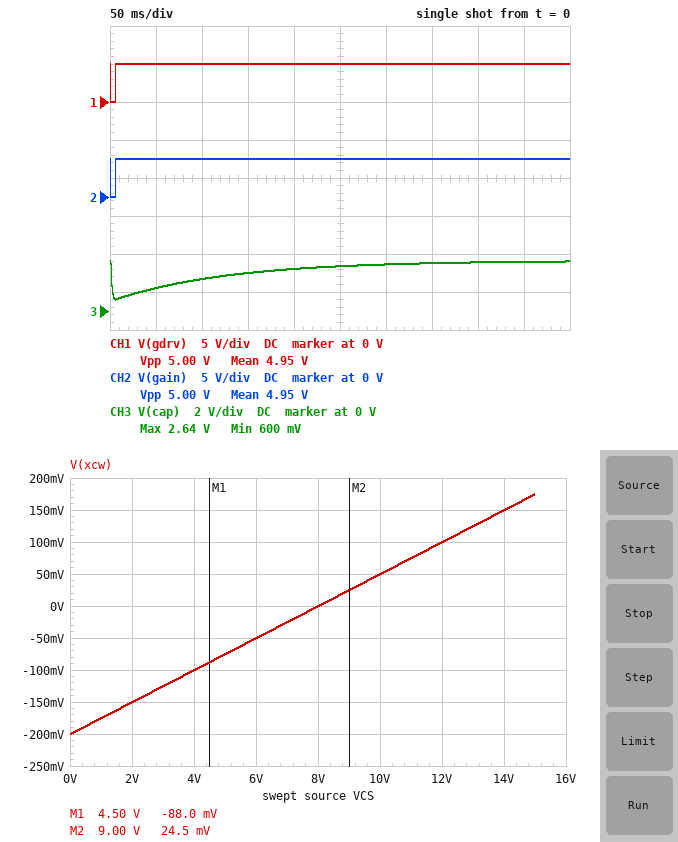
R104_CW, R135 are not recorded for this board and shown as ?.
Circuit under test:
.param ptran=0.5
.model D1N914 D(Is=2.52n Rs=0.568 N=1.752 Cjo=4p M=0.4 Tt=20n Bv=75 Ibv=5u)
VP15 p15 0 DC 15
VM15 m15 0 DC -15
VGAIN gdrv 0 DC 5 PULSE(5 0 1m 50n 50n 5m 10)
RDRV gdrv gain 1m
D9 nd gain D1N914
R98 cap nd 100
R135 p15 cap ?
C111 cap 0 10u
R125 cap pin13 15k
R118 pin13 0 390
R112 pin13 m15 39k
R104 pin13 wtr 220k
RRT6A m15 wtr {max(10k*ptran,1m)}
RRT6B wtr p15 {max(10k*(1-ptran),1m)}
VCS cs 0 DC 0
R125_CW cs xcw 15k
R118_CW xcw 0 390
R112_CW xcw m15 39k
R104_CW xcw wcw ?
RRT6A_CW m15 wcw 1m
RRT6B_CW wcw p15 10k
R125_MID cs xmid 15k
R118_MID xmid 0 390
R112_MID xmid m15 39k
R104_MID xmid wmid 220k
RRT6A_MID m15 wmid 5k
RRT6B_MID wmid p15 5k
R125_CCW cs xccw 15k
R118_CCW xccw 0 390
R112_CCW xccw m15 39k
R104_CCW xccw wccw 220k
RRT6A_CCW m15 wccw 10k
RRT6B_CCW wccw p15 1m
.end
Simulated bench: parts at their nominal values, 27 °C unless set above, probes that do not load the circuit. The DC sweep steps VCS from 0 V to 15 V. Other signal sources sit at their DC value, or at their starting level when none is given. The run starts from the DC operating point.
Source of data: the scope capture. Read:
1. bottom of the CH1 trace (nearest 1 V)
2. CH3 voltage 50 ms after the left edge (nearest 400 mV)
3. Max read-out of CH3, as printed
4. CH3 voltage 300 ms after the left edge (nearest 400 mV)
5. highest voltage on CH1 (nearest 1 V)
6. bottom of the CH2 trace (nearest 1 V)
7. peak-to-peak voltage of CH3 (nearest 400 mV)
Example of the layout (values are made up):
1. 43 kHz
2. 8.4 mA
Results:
1. 0 V
2. 1.2 V
3. 2.64 V
4. 2.4 V
5. 5 V
6. 0 V
7. 2.0 V
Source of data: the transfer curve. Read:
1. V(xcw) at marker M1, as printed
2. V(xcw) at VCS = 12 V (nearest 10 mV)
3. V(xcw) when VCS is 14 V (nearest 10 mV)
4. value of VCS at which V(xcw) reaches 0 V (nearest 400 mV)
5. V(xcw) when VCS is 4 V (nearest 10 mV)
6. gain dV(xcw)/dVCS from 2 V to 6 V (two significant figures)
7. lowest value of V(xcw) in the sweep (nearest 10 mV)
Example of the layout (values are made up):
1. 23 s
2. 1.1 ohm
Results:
1. -88.0 mV
2. 100 mV
3. 150 mV
4. 8.0 V
5. -100 mV
6. 0.025 V/V
7. -200 mV
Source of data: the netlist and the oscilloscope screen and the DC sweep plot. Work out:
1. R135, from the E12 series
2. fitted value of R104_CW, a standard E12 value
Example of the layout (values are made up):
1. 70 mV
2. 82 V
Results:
1. 68 kΩ
2. 100 kΩ
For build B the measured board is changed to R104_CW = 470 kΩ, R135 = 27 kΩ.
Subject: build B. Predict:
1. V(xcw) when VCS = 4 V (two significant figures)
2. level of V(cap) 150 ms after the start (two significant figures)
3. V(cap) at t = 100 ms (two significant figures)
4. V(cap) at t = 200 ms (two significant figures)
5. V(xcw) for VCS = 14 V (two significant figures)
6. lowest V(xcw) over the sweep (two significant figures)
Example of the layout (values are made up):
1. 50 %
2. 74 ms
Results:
1. -56 mV
2. 4.3 V
3. 3.6 V
4. 4.7 V
5. 190 mV
6. -160 mV
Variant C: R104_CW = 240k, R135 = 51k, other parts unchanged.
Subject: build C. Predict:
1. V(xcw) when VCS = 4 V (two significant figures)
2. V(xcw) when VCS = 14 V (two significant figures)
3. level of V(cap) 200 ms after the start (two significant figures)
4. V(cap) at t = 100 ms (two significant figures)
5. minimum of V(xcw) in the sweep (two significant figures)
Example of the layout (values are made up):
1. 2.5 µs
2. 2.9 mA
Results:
1. -68 mV
2. 180 mV
3. 2.8 V
4. 2.1 V
5. -170 mV
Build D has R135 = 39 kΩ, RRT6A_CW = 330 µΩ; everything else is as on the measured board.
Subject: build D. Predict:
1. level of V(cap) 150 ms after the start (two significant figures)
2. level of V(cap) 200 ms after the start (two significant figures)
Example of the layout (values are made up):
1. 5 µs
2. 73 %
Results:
1. 3.2 V
2. 3.5 V
